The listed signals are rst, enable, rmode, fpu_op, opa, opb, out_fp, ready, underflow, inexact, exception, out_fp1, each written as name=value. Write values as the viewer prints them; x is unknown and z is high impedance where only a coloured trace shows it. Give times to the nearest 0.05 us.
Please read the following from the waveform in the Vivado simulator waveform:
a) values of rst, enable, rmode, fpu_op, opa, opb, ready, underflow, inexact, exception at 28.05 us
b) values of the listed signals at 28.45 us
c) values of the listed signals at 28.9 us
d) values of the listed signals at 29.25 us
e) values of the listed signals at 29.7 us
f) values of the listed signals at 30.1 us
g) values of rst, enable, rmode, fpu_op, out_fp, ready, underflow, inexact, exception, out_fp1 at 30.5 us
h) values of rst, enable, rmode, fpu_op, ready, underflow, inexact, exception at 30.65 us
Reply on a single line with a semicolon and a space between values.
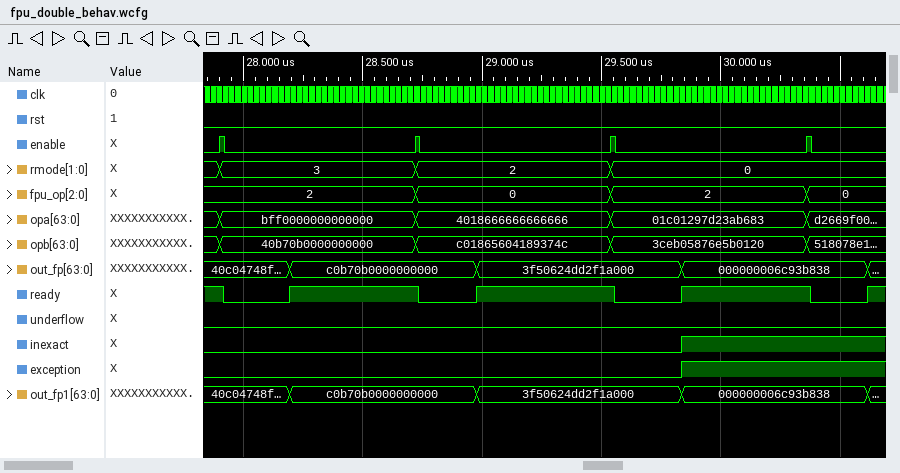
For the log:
rst=0, enable=0, rmode=3, fpu_op=2, opa=bff0000000000000, opb=40b70b0000000000, ready=0, underflow=0, inexact=0, exception=0; rst=0, enable=0, rmode=3, fpu_op=2, opa=bff0000000000000, opb=40b70b0000000000, out_fp=c0b70b0000000000, ready=1, underflow=0, inexact=0, exception=0, out_fp1=c0b70b0000000000; rst=0, enable=0, rmode=2, fpu_op=0, opa=4018666666666666, opb=c01865604189374c, out_fp=c0b70b0000000000, ready=0, underflow=0, inexact=0, exception=0, out_fp1=c0b70b0000000000; rst=0, enable=0, rmode=2, fpu_op=0, opa=4018666666666666, opb=c01865604189374c, out_fp=3f50624dd2f1a000, ready=1, underflow=0, inexact=0, exception=0, out_fp1=3f50624dd2f1a000; rst=0, enable=0, rmode=0, fpu_op=2, opa=01c01297d23ab683, opb=3ceb05876e5b0120, out_fp=3f50624dd2f1a000, ready=0, underflow=0, inexact=0, exception=0, out_fp1=3f50624dd2f1a000; rst=0, enable=0, rmode=0, fpu_op=2, opa=01c01297d23ab683, opb=3ceb05876e5b0120, out_fp=000000006c93b838, ready=1, underflow=0, inexact=1, exception=1, out_fp1=000000006c93b838; rst=0, enable=0, rmode=0, fpu_op=0, out_fp=000000006c93b838, ready=0, underflow=0, inexact=1, exception=1, out_fp1=000000006c93b838; rst=0, enable=0, rmode=0, fpu_op=0, ready=1, underflow=0, inexact=1, exception=1
